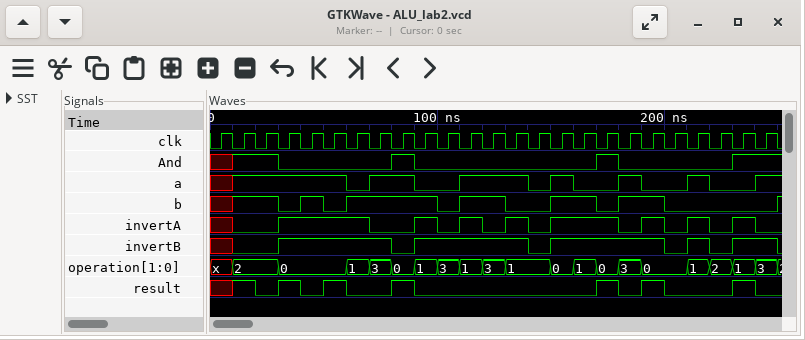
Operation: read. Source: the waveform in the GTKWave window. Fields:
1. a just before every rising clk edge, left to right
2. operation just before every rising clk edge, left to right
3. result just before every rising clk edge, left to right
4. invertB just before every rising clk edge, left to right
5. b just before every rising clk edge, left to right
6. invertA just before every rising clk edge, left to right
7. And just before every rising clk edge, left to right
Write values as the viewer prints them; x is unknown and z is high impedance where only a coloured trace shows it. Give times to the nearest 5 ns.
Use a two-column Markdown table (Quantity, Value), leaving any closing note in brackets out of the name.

| Quantity | Value |
|---|---|
| a just before every rising clk edge, left to right | x 1 1 1 1 1 0 1 1 0 0 1 1 1 0 1 0 0 1 0 0 1 0 0 1 |
| operation just before every rising clk edge, left to right | x, 2, 2, 0, 0, 0, 1, 3, 0, 1, 3, 1, 3, 1, 1, 0, 1, 0, 3, 0, 0, 1, 2, 1, 3 |
| result just before every rising clk edge, left to right | x 1 0 1 0 1 0 0 1 0 0 0 0 0 0 0 0 1 0 1 0 0 0 1 0 |
| invertB just before every rising clk edge, left to right | x 0 0 1 1 1 1 1 0 1 1 1 1 1 0 1 1 1 1 1 0 1 0 1 1 |
| b just before every rising clk edge, left to right | x 1 1 0 1 0 1 1 1 1 0 1 1 0 0 1 1 0 1 1 0 0 0 0 0 |
| invertA just before every rising clk edge, left to right | x 0 0 1 1 1 1 0 0 1 0 1 0 1 0 1 1 1 0 1 0 1 0 1 0 |
| And just before every rising clk edge, left to right | x 1 1 0 0 0 0 0 1 0 0 0 0 0 0 0 0 1 0 0 0 0 0 1 1 |
